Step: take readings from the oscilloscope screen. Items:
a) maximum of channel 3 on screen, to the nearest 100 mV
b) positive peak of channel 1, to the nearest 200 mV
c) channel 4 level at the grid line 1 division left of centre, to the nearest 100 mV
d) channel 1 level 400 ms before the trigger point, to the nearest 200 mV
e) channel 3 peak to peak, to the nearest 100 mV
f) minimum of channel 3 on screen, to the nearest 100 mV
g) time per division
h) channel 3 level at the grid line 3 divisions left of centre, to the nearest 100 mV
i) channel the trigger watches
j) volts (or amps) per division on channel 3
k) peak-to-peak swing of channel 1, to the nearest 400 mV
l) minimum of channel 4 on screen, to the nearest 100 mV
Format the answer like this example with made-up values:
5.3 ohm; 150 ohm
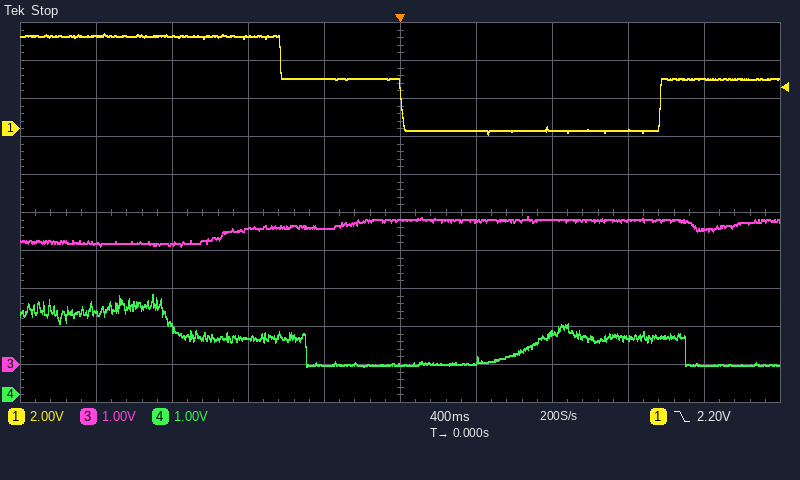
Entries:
3.9 V; 5.0 V; 800 mV; 2.6 V; 800 mV; 3.1 V; 400 ms; 3.2 V; channel 1; 1 V; 5.2 V; 700 mV
